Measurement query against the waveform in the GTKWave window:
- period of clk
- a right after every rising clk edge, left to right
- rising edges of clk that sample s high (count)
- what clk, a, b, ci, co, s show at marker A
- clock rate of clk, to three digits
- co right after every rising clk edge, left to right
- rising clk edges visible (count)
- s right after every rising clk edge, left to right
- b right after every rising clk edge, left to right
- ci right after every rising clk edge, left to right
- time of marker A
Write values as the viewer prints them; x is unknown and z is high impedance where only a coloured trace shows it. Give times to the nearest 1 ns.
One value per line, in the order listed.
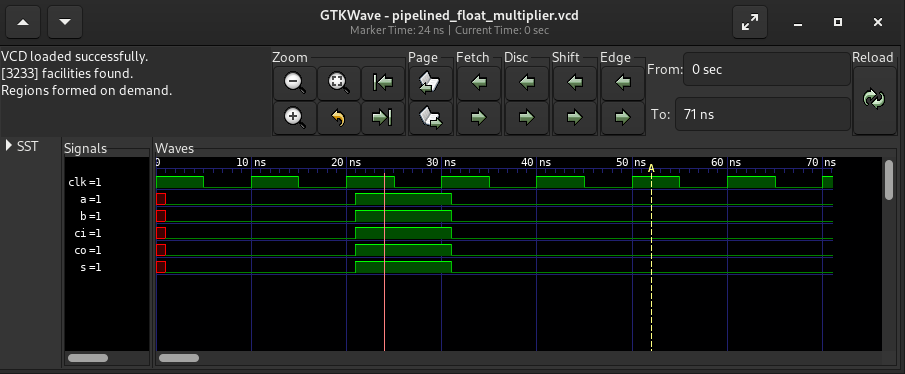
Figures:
10 ns
0 0 1 0 0 0 0
1
clk=1, a=0, b=0, ci=0, co=0, s=0
100 MHz
0 0 1 0 0 0 0
7
0 0 1 0 0 0 0
0 0 1 0 0 0 0
0 0 1 0 0 0 0
52 ns
